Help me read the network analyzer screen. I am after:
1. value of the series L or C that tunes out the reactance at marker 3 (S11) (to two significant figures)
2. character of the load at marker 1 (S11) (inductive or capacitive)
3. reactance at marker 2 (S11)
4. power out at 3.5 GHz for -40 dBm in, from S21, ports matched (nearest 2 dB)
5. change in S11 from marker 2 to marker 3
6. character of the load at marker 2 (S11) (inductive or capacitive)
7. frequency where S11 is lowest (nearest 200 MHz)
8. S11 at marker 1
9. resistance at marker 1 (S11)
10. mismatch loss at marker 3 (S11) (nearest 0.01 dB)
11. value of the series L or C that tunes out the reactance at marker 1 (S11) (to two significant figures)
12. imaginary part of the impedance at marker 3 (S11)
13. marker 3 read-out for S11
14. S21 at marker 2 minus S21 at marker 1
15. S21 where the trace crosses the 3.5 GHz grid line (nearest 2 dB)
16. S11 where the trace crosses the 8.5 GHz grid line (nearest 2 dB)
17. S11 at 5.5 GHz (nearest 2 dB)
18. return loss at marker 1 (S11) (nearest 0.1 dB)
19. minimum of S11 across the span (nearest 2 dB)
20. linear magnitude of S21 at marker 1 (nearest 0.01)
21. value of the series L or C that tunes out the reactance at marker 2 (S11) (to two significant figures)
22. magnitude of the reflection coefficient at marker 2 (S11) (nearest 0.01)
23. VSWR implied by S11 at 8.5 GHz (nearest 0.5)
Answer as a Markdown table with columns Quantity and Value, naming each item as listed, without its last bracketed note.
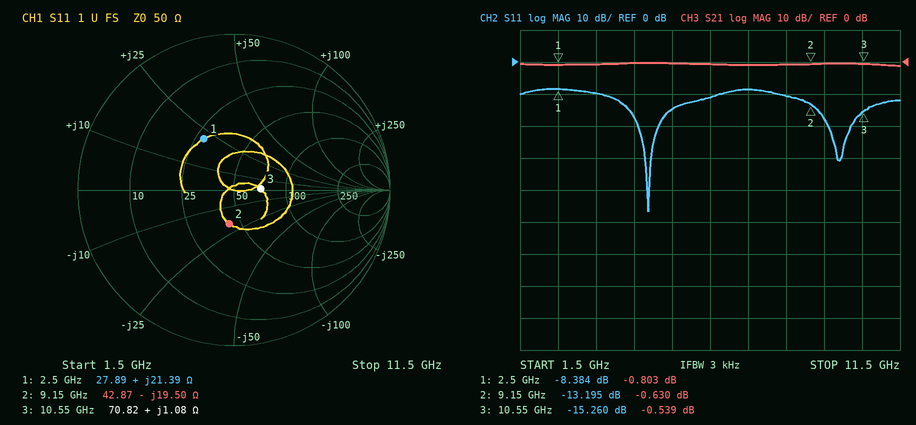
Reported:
| Quantity | Value |
|---|---|
| value of the series L or C that tunes out the reactance at marker 3 (S11) | 14 pF |
| character of the load at marker 1 (S11) | inductive |
| reactance at marker 2 | -19.50 Ω |
| power out at 3.5 GHz for -40 dBm in, from S21, ports matched | -40 dBm |
| change in S11 from marker 2 to marker 3 | -2.065 dB |
| character of the load at marker 2 (S11) | capacitive |
| frequency where S11 is lowest | 4.8 GHz |
| S11 at marker 1 | -8.384 dB |
| resistance at marker 1 | 27.89 Ω |
| mismatch loss at marker 3 (S11) | 0.13 dB |
| value of the series L or C that tunes out the reactance at marker 1 (S11) | 3.0 pF |
| imaginary part of the impedance at marker 3 | +1.08 Ω |
| marker 3 read-out for S11 | -15.260 dB |
| S21 at marker 2 minus S21 at marker 1 | 0.173 dB |
| S21 where the trace crosses the 3.5 GHz grid line | 0 dB |
| S11 where the trace crosses the 8.5 GHz grid line | -10 dB |
| S11 at 5.5 GHz | -14 dB |
| return loss at marker 1 (S11) | 8.4 dB |
| minimum of S11 across the span | -46 dB |
| linear magnitude of S21 at marker 1 | 0.91 |
| value of the series L or C that tunes out the reactance at marker 2 (S11) | 340 pH |
| magnitude of the reflection coefficient at marker 2 (S11) | 0.22 |
| VSWR implied by S11 at 8.5 GHz | 2.0 |
